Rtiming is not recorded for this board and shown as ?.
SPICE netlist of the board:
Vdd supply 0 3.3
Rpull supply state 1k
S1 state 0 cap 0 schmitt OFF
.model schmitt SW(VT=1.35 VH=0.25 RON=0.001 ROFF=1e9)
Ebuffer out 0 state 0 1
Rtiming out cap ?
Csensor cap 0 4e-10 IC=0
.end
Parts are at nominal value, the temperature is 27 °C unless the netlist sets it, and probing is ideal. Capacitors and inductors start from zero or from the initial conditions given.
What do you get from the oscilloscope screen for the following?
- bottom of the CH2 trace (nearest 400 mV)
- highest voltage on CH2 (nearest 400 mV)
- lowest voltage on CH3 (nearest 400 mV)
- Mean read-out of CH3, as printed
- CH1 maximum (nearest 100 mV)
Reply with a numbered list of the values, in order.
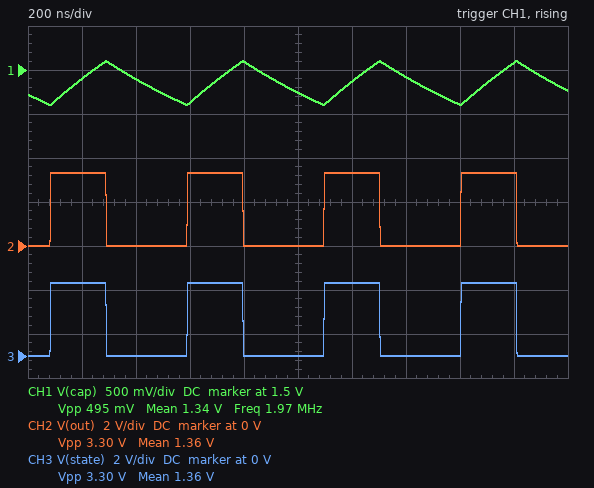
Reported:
1. 0 V
2. 3.2 V
3. 0 V
4. 1.36 V
5. 1.6 V
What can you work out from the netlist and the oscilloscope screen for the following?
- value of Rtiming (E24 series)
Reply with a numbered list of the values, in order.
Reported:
1. 2 kΩ
